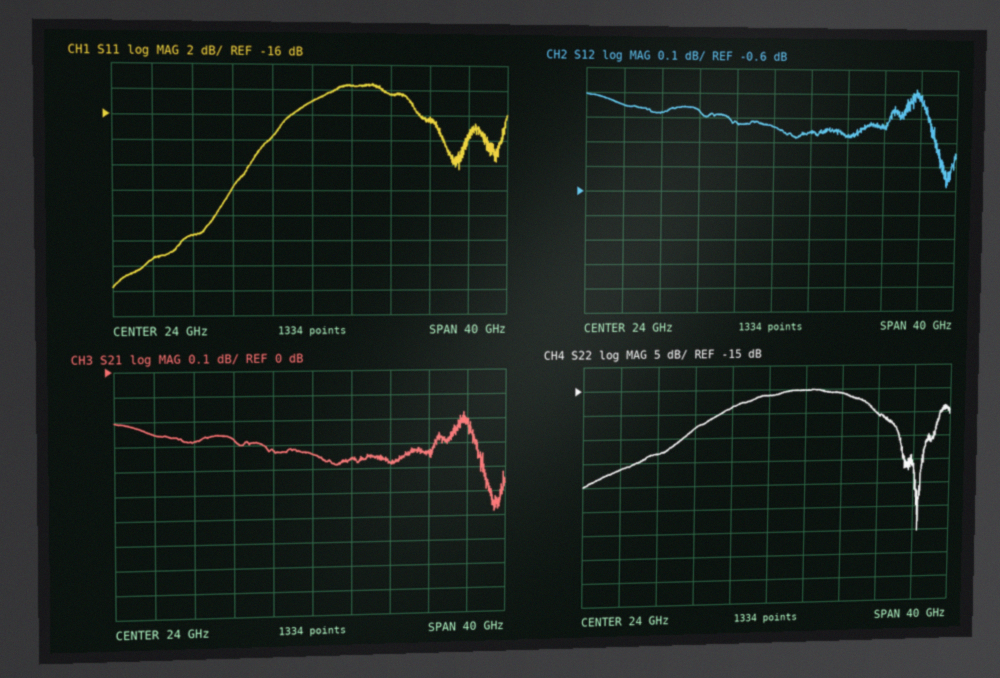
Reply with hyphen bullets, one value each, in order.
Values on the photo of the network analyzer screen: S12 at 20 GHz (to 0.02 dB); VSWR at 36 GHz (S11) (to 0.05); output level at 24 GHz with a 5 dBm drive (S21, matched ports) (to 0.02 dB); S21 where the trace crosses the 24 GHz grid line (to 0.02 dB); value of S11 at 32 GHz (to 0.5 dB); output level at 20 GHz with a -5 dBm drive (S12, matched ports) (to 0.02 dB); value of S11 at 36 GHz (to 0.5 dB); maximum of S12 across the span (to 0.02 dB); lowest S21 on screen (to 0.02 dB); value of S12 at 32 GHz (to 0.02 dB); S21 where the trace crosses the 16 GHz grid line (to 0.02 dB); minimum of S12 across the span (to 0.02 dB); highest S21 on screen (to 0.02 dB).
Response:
- -0.32 dB
- 1.35
- 4.66 dBm
- -0.34 dB
- -14.5 dB
- -5.32 dBm
- -16.5 dB
- -0.18 dB
- -0.58 dB
- -0.38 dB
- -0.28 dB
- -0.58 dB
- -0.18 dB
